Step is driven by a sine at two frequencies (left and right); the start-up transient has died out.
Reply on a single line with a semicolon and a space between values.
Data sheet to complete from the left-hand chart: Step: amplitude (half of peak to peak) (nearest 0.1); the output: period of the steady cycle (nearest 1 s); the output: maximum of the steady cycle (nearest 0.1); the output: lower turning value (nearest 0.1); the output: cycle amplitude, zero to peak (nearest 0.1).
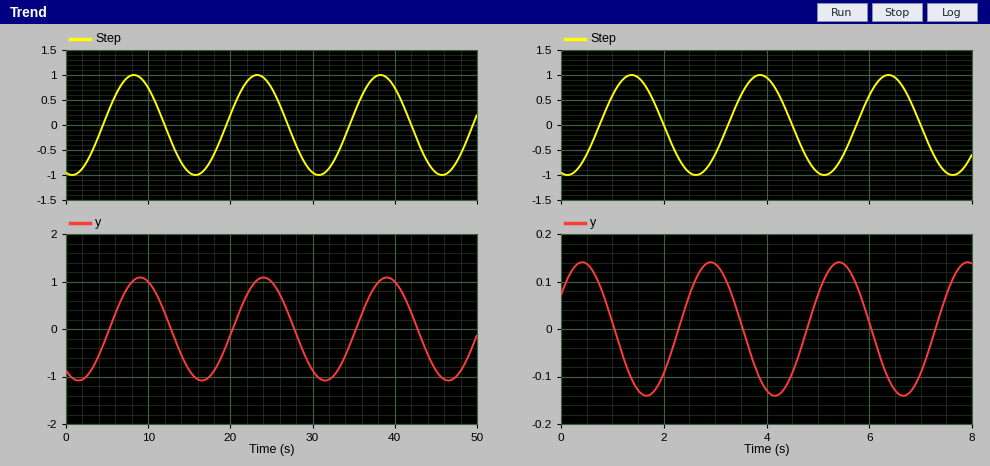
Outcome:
1.0; 15 s; 1.1; -1.1; 1.1
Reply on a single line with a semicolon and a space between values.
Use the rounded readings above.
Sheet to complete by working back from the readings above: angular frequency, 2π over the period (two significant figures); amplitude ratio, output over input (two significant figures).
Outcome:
0.42 rad/s; 1.1
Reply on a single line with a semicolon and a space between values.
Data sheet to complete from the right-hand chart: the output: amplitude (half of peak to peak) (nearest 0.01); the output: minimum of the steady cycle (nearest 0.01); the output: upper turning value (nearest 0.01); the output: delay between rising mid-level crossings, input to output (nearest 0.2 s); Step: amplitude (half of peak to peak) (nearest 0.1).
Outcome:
0.14; -0.14; 0.14; 1.6 s; 1.0
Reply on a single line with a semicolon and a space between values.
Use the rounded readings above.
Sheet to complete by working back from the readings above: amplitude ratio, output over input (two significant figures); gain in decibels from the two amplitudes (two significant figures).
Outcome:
0.14; -17 dB
